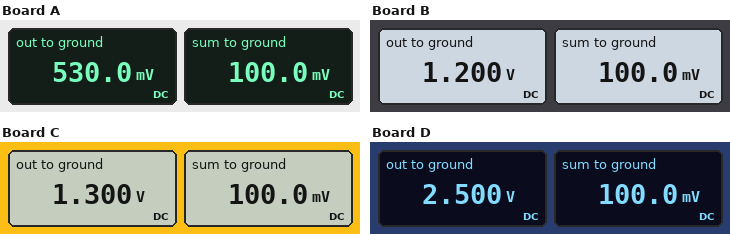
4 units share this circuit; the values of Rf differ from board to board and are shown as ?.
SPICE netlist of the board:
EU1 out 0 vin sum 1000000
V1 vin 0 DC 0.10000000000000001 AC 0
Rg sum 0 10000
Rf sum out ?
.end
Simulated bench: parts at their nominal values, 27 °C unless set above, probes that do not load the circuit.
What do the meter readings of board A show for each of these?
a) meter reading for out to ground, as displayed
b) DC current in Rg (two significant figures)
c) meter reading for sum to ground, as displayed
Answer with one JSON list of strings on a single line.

["530.0 mV", "10 µA", "100.0 mV"]
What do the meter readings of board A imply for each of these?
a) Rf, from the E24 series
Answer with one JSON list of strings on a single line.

["43 kΩ"]
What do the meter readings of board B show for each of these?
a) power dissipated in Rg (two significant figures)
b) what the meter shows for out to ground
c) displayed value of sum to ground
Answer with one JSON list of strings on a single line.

["1.0 µW", "1.200 V", "100.0 mV"]
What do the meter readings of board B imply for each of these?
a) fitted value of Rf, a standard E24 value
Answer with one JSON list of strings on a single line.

["110 kΩ"]
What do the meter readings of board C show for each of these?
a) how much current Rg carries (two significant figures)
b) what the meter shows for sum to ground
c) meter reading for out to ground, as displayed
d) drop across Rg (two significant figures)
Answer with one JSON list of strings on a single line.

["10 µA", "100.0 mV", "1.300 V", "100 mV"]
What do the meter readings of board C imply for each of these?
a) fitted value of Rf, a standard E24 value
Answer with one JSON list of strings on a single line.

["120 kΩ"]
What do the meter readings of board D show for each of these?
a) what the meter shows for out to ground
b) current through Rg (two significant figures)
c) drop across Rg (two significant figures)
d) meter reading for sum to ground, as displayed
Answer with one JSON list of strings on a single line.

["2.500 V", "10 µA", "100 mV", "100.0 mV"]
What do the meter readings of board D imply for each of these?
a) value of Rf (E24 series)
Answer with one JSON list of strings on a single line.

["240 kΩ"]
